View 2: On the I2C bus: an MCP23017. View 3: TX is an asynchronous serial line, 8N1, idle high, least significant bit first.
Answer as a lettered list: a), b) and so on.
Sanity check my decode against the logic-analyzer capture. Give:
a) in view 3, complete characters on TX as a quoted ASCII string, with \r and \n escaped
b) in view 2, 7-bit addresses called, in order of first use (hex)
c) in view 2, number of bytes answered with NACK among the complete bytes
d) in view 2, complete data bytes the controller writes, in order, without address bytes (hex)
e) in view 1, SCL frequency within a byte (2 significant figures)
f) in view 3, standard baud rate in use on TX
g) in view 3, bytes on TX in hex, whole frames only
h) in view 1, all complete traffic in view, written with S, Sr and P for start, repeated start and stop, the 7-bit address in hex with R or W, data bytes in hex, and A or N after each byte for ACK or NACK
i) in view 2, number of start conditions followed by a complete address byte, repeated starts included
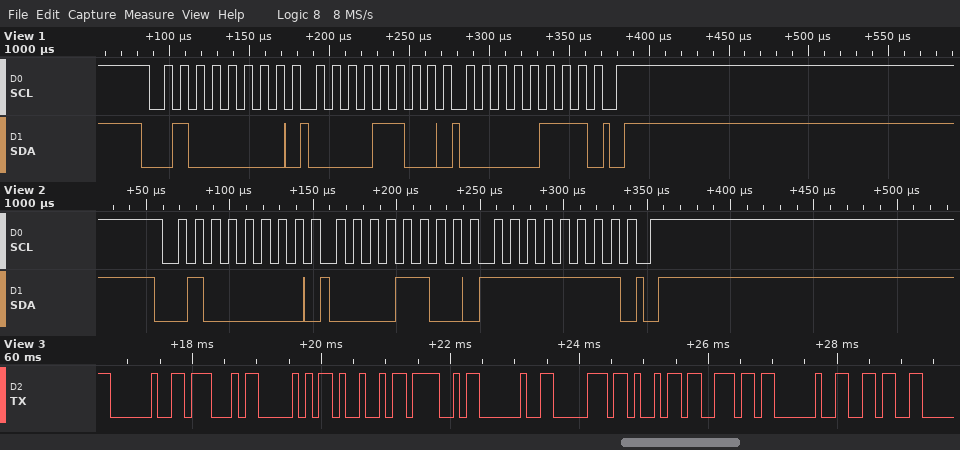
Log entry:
a) " GPIO pin 6"
b) 0x20
c) 0
d) 0C FF
e) 100 kHz
f) 9600 baud
g) 20 47 50 49 4F 20 70 69 6E 20 36
h) S 20W A 0C A 07 A P
i) 1
